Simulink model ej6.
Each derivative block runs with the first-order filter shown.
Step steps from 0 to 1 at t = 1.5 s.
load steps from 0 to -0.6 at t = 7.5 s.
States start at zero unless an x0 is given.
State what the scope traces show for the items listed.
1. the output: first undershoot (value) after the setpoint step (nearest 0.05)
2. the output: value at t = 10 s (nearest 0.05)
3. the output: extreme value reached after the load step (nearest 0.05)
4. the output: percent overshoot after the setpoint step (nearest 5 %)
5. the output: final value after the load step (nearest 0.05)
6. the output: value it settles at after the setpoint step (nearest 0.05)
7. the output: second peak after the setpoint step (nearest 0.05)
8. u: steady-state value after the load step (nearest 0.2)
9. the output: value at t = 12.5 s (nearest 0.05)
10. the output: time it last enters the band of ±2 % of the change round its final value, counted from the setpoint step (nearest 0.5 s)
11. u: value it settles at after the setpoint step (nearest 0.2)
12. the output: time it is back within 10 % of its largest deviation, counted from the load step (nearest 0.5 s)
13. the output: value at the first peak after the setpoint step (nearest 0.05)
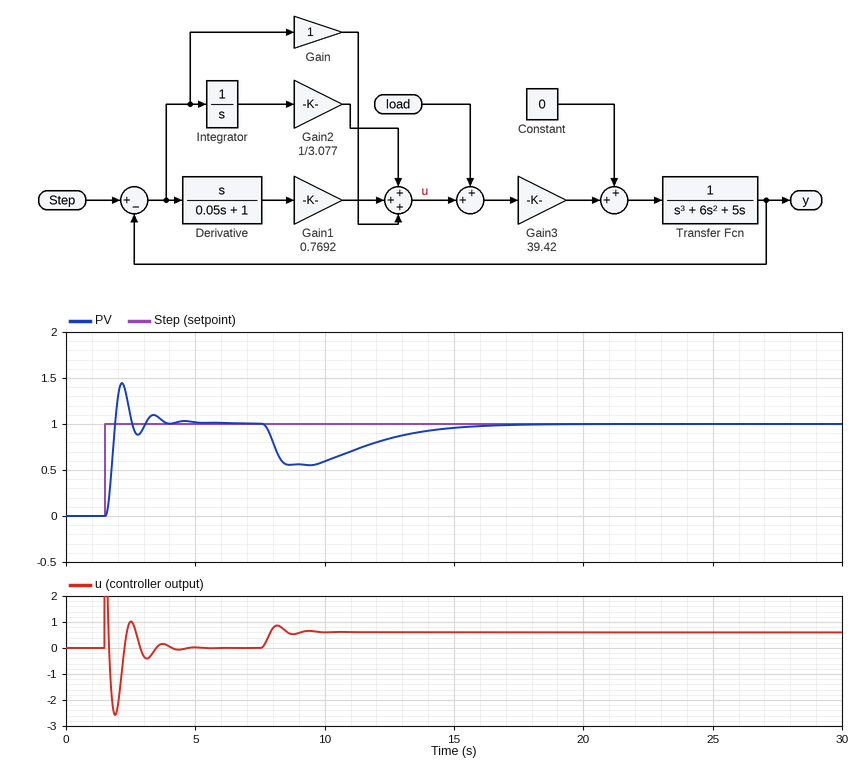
0.90
0.60
0.55
45 %
1.00
1.00
1.10
0.6
0.85
3.5 s
0.0
7.5 s
1.45
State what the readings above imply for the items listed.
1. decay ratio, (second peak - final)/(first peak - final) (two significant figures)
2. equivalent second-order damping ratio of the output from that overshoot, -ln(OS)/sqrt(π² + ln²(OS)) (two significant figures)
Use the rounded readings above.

0.22
0.25
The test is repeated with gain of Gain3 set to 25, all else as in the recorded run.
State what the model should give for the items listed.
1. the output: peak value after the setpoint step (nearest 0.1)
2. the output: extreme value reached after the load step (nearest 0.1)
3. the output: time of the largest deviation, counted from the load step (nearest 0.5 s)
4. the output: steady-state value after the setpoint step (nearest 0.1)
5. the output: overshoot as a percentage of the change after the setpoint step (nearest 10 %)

1.3
0.5
1.5 s
1.0
30 %
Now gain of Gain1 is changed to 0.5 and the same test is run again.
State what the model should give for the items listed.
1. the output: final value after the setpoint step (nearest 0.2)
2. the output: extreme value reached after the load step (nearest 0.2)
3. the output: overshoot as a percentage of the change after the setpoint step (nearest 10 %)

1.0
0.4
50 %
